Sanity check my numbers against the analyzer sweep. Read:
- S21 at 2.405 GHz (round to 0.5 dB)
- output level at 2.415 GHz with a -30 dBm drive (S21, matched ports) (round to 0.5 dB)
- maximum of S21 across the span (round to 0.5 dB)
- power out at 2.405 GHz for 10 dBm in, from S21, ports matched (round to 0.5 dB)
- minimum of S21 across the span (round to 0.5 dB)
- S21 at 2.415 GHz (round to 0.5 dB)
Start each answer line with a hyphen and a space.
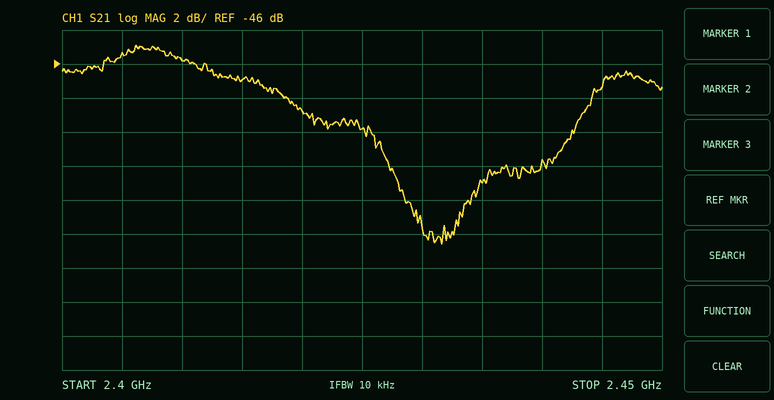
- -45.5 dB
- -77.0 dBm
- -45.0 dB
- -35.5 dBm
- -56.5 dB
- -47.0 dB
